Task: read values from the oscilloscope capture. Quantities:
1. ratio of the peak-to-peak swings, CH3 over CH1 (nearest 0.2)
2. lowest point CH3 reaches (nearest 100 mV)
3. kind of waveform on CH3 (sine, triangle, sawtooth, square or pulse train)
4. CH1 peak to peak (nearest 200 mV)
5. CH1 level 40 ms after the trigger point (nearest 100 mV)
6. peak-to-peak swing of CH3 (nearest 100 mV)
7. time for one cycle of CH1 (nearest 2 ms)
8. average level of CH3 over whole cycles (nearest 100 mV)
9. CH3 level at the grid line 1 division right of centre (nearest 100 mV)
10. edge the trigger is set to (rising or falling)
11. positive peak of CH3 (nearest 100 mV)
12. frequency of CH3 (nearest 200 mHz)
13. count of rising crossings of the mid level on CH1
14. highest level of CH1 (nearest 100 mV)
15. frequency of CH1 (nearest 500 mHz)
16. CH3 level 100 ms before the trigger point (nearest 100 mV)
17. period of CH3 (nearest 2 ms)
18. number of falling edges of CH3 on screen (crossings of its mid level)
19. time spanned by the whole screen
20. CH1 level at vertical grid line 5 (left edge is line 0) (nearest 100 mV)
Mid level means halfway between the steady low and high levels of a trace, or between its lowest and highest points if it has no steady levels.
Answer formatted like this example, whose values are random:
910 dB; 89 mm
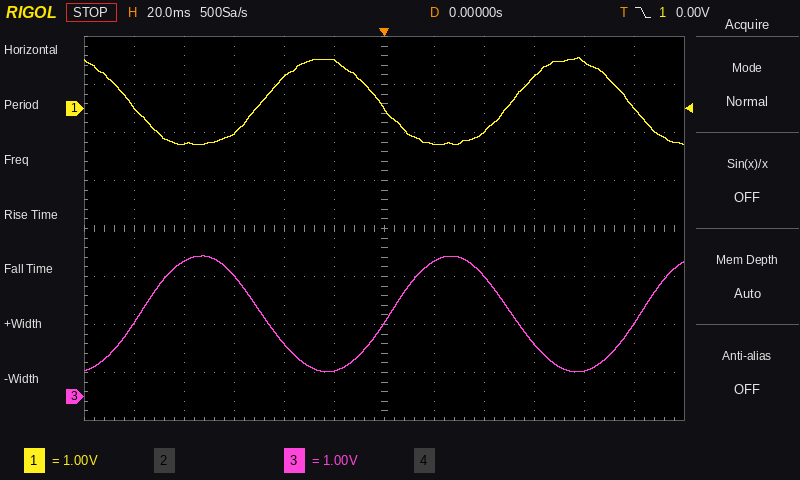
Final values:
1.4; 500 mV; sine; 1.8 V; -500 mV; 2.4 V; 100 ms; 1.7 V; 2.8 V; falling; 2.9 V; 10.0 Hz; 2; 1.1 V; 10.0 Hz; 1.5 V; 100 ms; 2; 240 ms; 1.0 V
